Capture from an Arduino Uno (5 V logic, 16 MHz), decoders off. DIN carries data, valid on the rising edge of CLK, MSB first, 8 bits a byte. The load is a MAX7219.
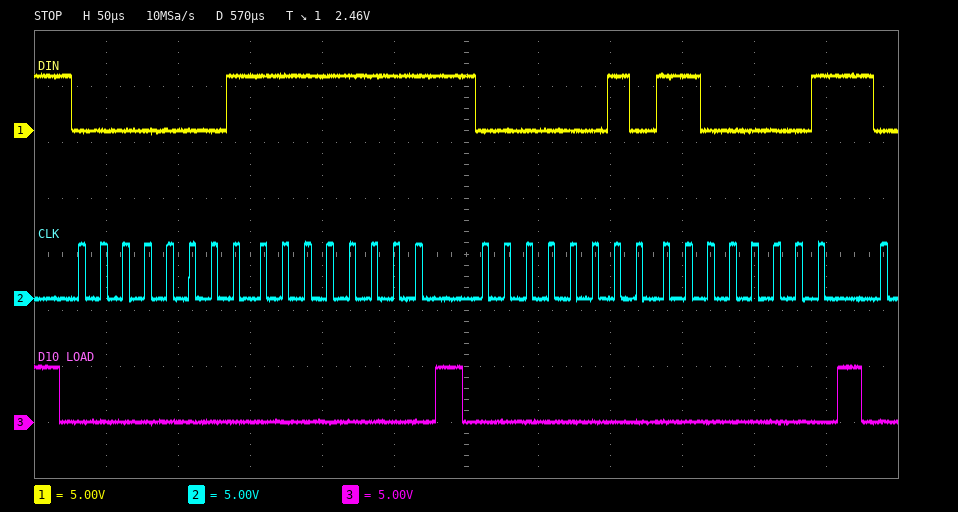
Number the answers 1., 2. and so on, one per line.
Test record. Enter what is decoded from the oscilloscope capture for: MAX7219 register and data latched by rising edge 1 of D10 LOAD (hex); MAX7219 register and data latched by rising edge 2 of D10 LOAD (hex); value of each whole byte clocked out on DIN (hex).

1. register 0x1, data 0xFF
2. register 0x2, data 0xC1
3. 0x01 0xFF 0x02 0xC1
